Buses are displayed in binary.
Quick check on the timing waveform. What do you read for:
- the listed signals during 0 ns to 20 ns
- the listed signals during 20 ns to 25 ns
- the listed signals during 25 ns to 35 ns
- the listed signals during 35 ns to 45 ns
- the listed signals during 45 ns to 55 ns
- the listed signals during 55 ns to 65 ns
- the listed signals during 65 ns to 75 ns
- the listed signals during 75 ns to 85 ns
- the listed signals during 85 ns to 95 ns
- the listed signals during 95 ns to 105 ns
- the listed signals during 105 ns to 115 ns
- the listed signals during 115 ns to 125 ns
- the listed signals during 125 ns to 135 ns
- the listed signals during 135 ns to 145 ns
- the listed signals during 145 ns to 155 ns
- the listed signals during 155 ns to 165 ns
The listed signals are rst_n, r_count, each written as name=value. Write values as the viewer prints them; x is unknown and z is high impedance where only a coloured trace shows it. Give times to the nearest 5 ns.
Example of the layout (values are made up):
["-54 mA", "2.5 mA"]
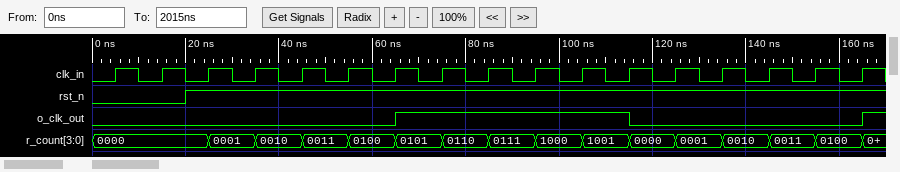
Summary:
["rst_n=0, r_count=0000", "rst_n=1, r_count=0000", "rst_n=1, r_count=0001", "rst_n=1, r_count=0010", "rst_n=1, r_count=0011", "rst_n=1, r_count=0100", "rst_n=1, r_count=0101", "rst_n=1, r_count=0110", "rst_n=1, r_count=0111", "rst_n=1, r_count=1000", "rst_n=1, r_count=1001", "rst_n=1, r_count=0000", "rst_n=1, r_count=0001", "rst_n=1, r_count=0010", "rst_n=1, r_count=0011", "rst_n=1, r_count=0100"]
